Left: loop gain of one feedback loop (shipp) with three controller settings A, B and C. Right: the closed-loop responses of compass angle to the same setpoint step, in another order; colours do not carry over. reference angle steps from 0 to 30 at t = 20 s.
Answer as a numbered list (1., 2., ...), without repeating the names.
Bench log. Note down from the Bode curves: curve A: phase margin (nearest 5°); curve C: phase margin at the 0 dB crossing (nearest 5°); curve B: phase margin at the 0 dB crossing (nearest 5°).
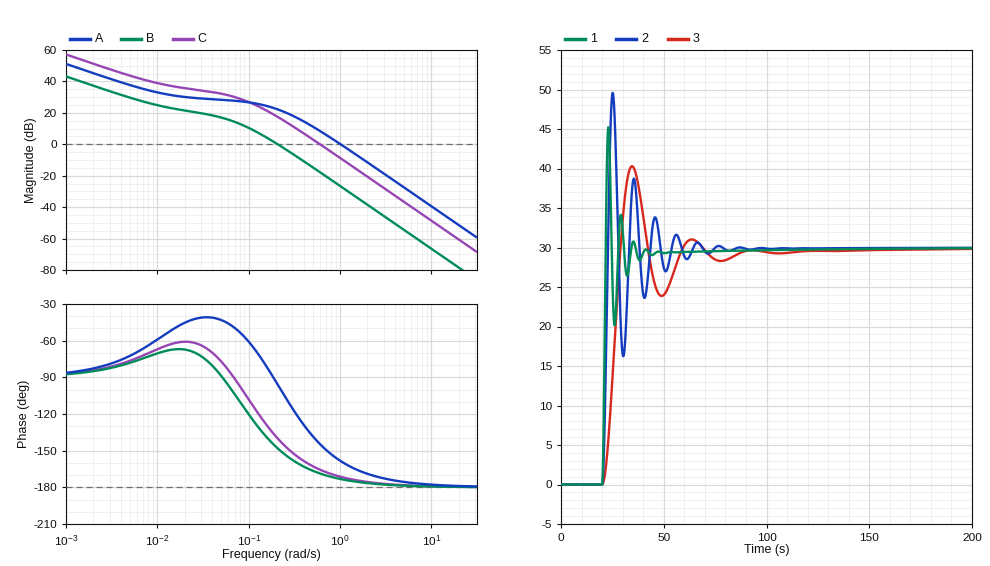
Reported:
1. 20°
2. 15°
3. 30°
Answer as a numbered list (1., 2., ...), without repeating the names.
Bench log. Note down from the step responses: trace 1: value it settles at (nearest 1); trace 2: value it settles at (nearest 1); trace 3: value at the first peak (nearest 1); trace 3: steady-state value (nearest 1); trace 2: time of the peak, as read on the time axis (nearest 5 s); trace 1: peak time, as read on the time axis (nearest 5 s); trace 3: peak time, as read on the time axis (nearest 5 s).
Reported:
1. 30
2. 30
3. 40
4. 30
5. 25 s
6. 25 s
7. 35 s
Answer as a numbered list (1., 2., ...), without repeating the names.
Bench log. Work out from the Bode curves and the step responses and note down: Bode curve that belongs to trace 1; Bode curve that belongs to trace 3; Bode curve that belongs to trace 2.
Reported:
1. A
2. B
3. C
